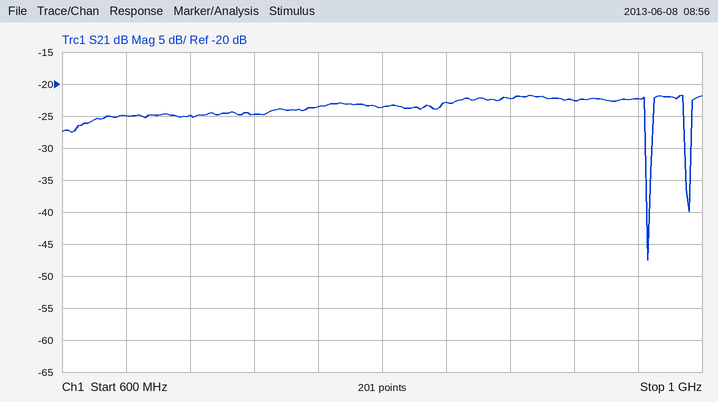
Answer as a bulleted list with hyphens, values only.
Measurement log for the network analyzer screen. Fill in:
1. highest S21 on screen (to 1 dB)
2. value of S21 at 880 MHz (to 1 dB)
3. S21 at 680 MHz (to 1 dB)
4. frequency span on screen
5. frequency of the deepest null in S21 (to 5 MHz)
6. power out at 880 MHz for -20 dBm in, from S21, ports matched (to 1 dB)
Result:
- -22 dB
- -22 dB
- -25 dB
- 400 MHz
- 965 MHz
- -42 dBm
